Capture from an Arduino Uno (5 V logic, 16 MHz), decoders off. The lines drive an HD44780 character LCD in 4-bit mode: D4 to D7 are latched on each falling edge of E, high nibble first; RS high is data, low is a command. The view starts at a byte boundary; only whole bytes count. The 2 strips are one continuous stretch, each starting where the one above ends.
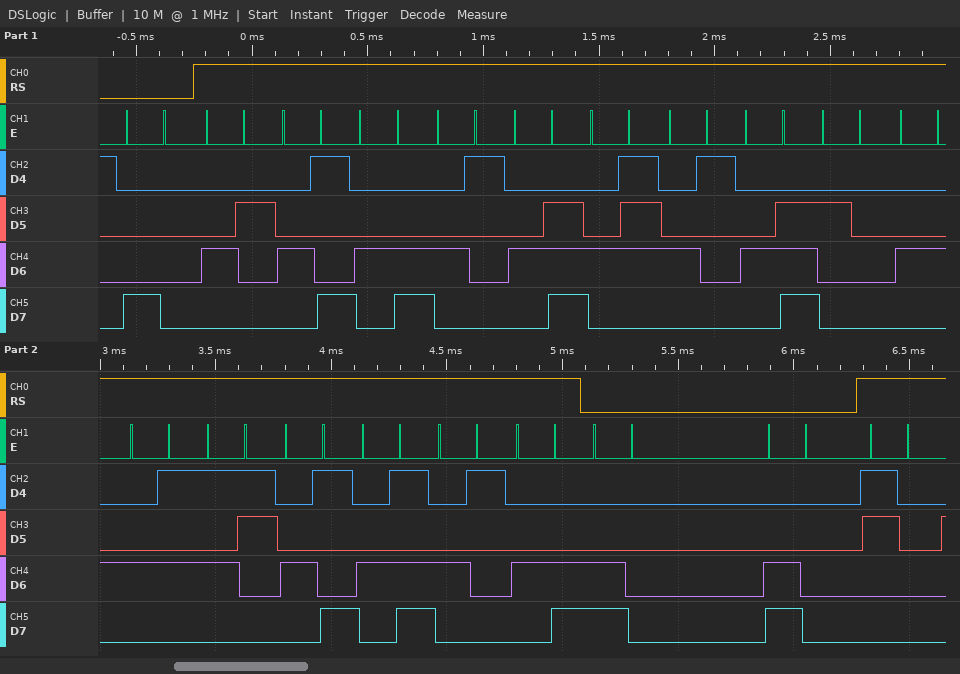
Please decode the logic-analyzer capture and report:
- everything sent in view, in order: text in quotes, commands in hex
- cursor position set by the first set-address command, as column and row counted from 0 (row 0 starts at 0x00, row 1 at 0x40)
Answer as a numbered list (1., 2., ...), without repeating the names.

1. 0x80 "BILANGAN DESIMAL" 0xC0 0xC0 "0"
2. column 0, row 0
